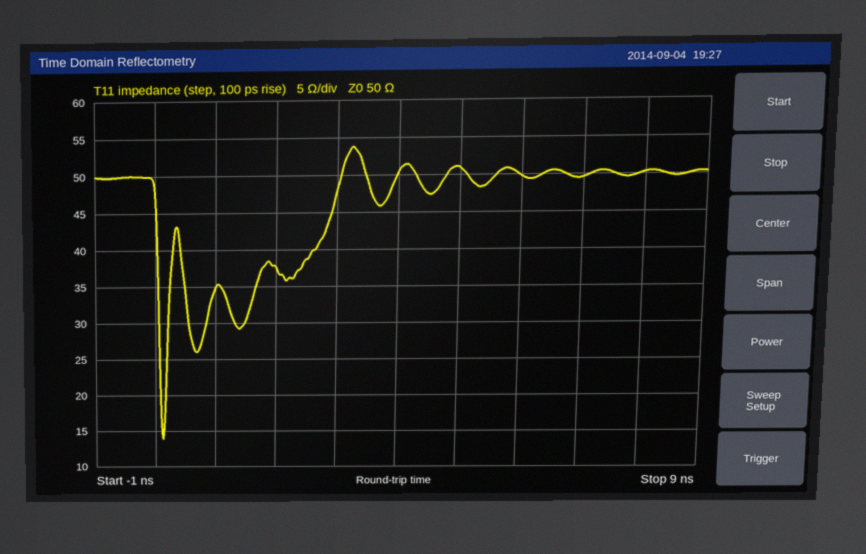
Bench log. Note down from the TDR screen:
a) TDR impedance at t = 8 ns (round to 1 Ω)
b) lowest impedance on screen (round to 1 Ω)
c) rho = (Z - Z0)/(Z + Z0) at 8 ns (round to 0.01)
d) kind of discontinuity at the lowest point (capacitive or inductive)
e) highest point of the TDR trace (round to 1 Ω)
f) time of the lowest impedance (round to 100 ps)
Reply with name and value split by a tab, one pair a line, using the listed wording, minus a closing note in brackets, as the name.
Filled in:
TDR impedance at t = 8 ns	50 Ω
lowest impedance on screen	14 Ω
rho = (Z - Z0)/(Z + Z0) at 8 ns	0.00
kind of discontinuity at the lowest point	capacitive
highest point of the TDR trace	54 Ω
time of the lowest impedance	100 ps
